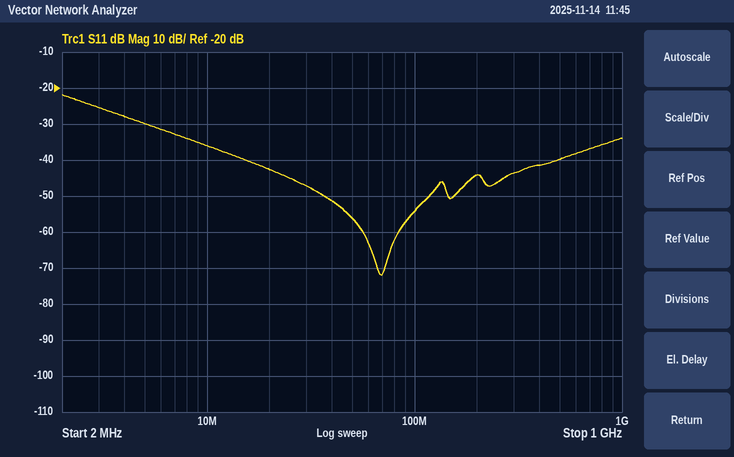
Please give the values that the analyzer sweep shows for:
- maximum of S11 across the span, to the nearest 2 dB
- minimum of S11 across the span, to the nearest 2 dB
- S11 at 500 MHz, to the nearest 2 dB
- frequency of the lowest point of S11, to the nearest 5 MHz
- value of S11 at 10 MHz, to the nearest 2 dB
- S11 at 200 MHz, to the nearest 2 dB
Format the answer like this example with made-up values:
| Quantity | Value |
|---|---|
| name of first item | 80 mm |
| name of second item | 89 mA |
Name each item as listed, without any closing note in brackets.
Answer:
| Quantity | Value |
|---|---|
| maximum of S11 across the span, to the nearest 2 dB | -22 dB |
| minimum of S11 across the span, to the nearest 2 dB | -72 dB |
| S11 at 500 MHz, to the nearest 2 dB | -40 dB |
| frequency of the lowest point of S11, to the nearest 5 MHz | 70 MHz |
| value of S11 at 10 MHz, to the nearest 2 dB | -36 dB |
| S11 at 200 MHz, to the nearest 2 dB | -44 dB |
